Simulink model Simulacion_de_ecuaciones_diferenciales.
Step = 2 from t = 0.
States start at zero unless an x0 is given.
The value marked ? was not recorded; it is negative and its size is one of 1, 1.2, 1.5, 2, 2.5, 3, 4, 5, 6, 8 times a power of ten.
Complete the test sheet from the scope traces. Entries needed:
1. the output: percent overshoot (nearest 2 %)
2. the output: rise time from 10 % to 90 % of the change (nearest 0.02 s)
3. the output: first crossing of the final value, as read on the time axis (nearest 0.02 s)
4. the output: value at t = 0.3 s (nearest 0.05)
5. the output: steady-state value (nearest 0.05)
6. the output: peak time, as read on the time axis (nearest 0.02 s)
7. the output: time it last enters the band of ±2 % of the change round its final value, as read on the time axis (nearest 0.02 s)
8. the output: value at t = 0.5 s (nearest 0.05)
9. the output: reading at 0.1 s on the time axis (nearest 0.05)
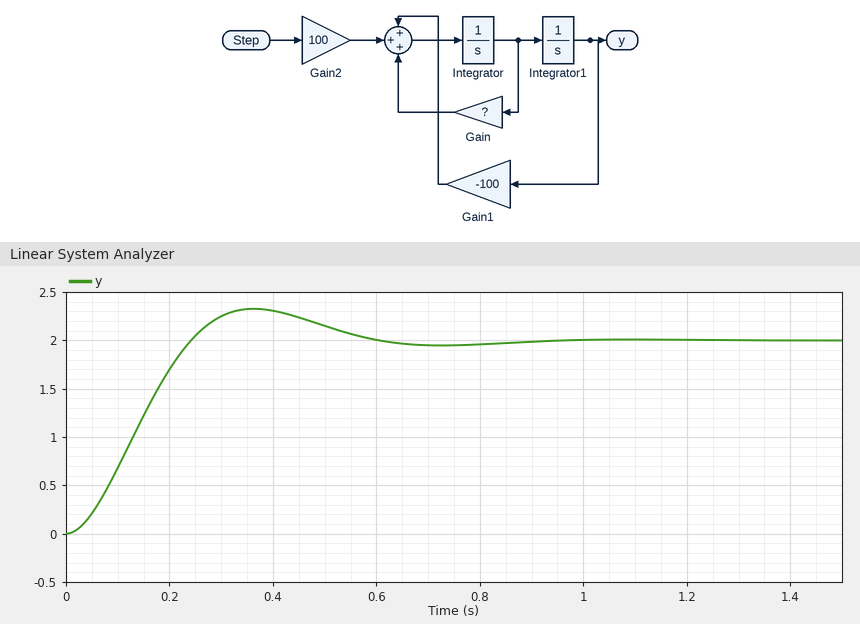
16 %
0.16 s
0.24 s
2.25
2.00
0.36 s
0.80 s
2.15
0.70
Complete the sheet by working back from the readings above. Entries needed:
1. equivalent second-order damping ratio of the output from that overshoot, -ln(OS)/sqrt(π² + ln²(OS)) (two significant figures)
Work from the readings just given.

0.50
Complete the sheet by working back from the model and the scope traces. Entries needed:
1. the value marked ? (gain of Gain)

-10
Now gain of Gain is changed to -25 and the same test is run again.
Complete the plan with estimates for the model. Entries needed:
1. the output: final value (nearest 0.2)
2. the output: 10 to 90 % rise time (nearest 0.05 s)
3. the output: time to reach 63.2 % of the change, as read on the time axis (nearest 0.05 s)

2.0
0.45 s
0.25 s
